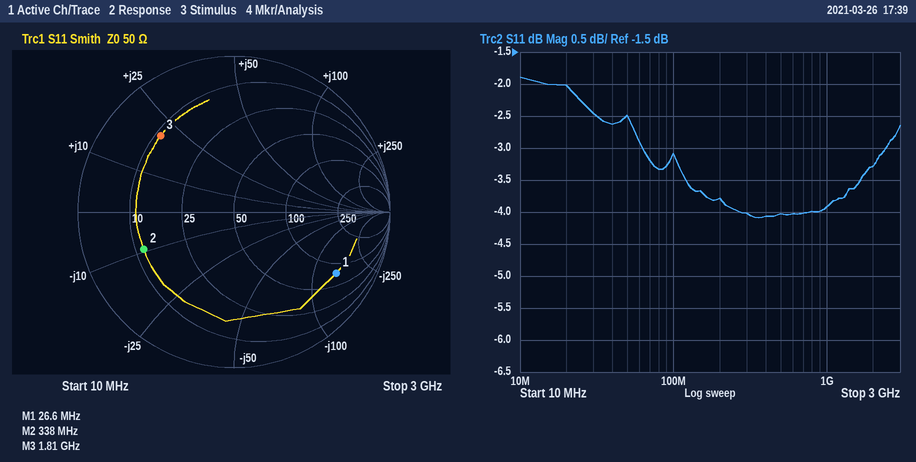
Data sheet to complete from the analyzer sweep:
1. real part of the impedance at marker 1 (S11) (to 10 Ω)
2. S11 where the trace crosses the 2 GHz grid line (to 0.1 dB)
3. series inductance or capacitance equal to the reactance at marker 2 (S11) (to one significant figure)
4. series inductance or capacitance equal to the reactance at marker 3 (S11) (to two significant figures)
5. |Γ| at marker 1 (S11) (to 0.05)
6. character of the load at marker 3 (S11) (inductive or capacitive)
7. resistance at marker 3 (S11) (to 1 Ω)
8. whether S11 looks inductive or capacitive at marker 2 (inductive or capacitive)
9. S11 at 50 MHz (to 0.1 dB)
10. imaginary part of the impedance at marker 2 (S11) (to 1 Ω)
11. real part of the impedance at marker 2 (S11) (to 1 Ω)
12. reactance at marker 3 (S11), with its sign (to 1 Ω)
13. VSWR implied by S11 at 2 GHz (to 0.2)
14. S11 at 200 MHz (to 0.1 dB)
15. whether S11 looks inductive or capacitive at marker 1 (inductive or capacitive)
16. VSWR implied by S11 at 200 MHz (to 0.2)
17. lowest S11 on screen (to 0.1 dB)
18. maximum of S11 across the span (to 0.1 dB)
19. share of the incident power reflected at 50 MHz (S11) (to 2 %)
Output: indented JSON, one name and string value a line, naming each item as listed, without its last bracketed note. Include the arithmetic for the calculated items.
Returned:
{
  "real part of the impedance at marker 1 (S11)": "80 Ω",
  "S11 where the trace crosses the 2 GHz grid line": "-3.3 dB",
  "series inductance or capacitance equal to the reactance at marker 2 (S11)": "C = 1/(2π × 338 MHz × 9 Ω) ≈ 52.3 pF, so 50 pF to one significant figure",
  "series inductance or capacitance equal to the reactance at marker 3 (S11)": "L = 20 Ω/(2π × 1.81 GHz) ≈ 1.8 nH",
  "|Γ| at marker 1 (S11)": "0.75",
  "character of the load at marker 3 (S11)": "inductive",
  "resistance at marker 3 (S11)": "11 Ω",
  "whether S11 looks inductive or capacitive at marker 2": "capacitive",
  "S11 at 50 MHz": "-2.5 dB",
  "imaginary part of the impedance at marker 2 (S11)": "-9 Ω",
  "real part of the impedance at marker 2 (S11)": "12 Ω",
  "reactance at marker 3 (S11), with its sign": "+20 Ω",
  "VSWR implied by S11 at 2 GHz": "|Γ| = 10^(-3.3/20) = 0.6839; VSWR = (1 + 0.6839)/(1 − 0.6839) ≈ 5.33, so 5.4 to the nearest 0.2",
  "S11 at 200 MHz": "-3.8 dB",
  "whether S11 looks inductive or capacitive at marker 1": "capacitive",
  "VSWR implied by S11 at 200 MHz": "|Γ| = 10^(-3.8/20) = 0.6457; VSWR = (1 + 0.6457)/(1 − 0.6457) ≈ 4.6",
  "lowest S11 on screen": "-4.1 dB",
  "maximum of S11 across the span": "-1.9 dB",
  "share of the incident power reflected at 50 MHz (S11)": "10^(-2.5/10) ≈ 56 %"
}
